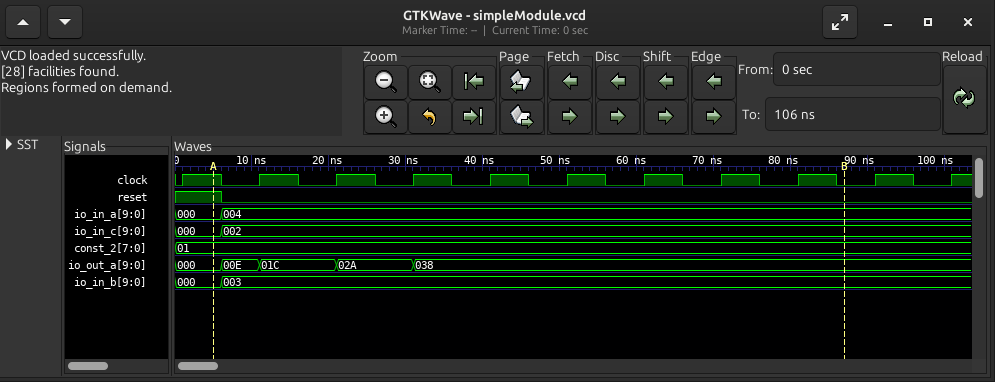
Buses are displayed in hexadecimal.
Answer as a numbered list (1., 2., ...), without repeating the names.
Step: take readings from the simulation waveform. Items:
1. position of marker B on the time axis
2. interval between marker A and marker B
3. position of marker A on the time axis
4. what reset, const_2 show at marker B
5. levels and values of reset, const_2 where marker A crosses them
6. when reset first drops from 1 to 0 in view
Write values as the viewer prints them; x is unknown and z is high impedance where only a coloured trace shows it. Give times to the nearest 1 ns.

1. 87 ns
2. 82 ns
3. 5 ns
4. reset=0, const_2=01
5. reset=1, const_2=01
6. 6 ns
